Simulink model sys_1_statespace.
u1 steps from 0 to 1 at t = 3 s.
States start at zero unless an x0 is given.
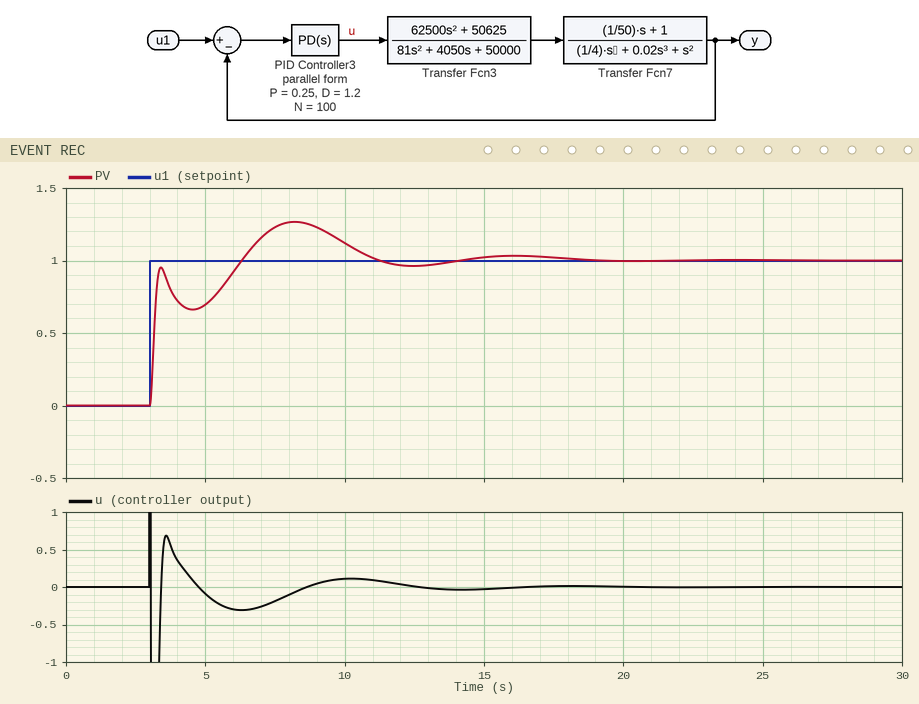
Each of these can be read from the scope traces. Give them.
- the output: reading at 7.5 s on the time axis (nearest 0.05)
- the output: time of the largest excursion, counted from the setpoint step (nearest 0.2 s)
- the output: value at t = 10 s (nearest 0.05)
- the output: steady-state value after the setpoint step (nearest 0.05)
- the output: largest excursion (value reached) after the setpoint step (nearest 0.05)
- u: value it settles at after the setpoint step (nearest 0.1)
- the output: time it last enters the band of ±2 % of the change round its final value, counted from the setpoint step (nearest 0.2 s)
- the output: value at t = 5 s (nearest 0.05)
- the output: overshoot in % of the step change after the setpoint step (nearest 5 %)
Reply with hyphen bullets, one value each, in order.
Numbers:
- 1.25
- 5.2 s
- 1.10
- 1.00
- 1.25
- 0.0
- 14.6 s
- 0.70
- 25 %
